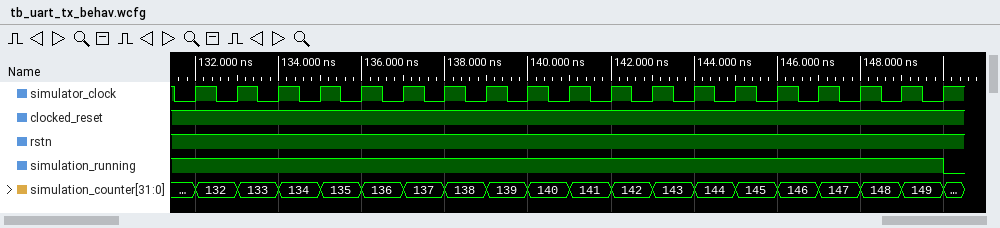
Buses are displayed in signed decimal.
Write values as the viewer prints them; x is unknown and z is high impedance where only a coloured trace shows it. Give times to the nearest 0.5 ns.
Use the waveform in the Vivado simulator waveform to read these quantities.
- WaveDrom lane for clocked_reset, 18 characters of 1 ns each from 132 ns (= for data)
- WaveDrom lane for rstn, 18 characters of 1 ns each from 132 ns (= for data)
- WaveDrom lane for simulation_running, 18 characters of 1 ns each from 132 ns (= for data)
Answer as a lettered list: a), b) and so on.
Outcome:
a) {name: 'clocked_reset', wave: '1.................'}
b) {name: 'rstn', wave: '1.................'}
c) {name: 'simulation_running', wave: '1.................'}
